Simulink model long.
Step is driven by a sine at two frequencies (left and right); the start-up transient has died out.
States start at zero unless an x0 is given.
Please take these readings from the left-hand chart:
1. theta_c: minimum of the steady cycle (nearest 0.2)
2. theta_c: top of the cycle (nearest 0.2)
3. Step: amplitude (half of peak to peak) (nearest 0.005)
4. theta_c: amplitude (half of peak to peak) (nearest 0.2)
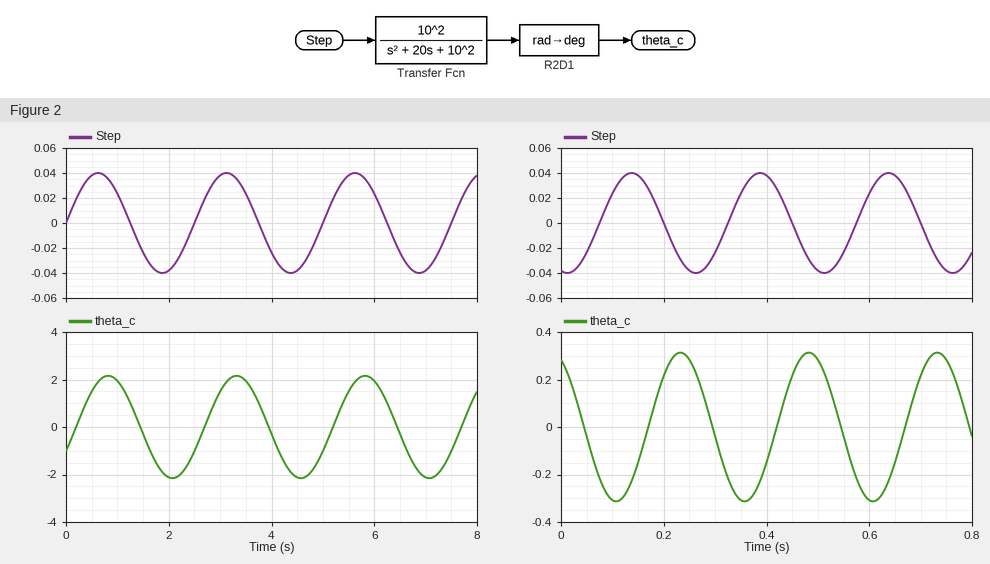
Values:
-2.2
2.2
0.040
2.2
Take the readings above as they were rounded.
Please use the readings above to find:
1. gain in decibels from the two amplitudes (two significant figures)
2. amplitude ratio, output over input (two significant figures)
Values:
35 dB
55
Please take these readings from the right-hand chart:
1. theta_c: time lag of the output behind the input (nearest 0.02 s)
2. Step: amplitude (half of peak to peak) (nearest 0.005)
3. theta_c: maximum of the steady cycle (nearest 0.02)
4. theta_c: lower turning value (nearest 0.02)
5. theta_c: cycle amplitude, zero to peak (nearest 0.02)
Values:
0.10 s
0.040
0.32
-0.32
0.32
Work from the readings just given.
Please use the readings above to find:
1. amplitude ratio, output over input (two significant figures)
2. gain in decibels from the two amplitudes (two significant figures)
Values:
8.0
18 dB
